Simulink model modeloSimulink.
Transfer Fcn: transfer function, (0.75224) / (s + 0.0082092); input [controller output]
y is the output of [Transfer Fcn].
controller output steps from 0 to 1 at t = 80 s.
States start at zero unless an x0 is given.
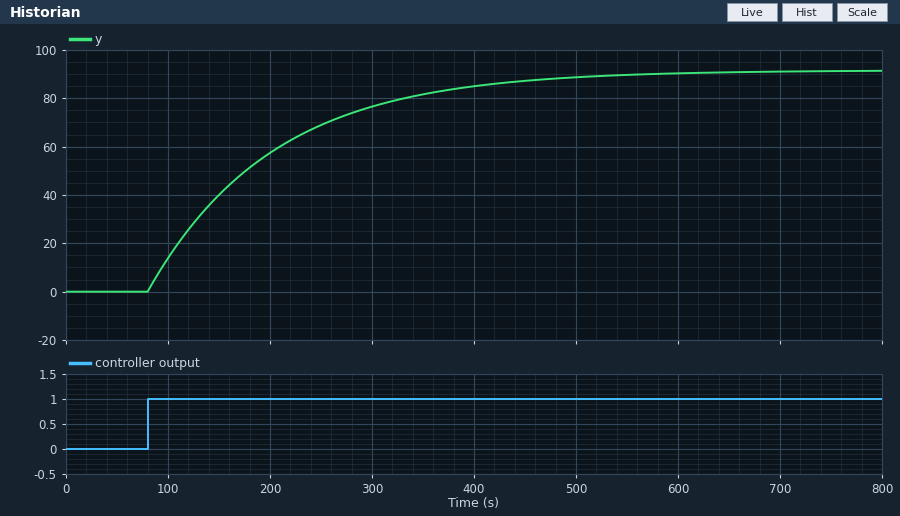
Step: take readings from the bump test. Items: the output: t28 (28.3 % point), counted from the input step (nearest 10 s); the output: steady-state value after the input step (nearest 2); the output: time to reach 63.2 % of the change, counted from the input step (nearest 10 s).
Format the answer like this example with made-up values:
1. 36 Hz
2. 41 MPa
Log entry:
1. 40 s
2. 92
3. 120 s
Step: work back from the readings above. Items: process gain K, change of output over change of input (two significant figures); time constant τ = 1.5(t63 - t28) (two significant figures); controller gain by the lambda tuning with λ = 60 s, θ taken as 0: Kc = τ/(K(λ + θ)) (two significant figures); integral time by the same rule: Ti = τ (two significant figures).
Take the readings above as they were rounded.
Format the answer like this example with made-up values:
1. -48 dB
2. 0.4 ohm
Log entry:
1. 92
2. 120 s
3. 0.022
4. 120 s
